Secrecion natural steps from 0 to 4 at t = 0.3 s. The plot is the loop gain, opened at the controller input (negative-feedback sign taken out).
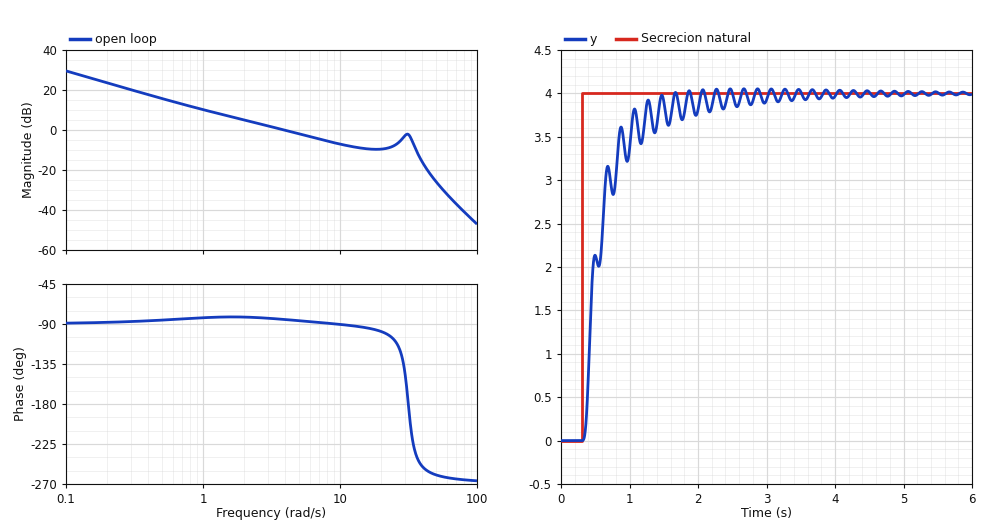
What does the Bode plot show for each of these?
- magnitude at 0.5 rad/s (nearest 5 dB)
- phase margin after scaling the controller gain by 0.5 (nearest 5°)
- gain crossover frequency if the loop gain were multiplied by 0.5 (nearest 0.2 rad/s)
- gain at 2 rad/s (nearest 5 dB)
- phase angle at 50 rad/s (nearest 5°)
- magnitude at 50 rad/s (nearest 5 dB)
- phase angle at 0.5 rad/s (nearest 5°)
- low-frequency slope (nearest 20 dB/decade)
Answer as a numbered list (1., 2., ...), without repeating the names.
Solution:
1. 15 dB
2. 100°
3. 1.8 rad/s
4. 5 dB
5. -260°
6. -25 dB
7. -85°
8. -20 dB/decade
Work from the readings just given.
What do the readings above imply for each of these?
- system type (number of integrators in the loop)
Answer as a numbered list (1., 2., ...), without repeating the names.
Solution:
1. 1
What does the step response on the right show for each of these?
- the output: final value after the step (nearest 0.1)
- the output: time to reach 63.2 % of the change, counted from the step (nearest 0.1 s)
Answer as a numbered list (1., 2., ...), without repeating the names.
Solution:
1. 4.0
2. 0.3 s
